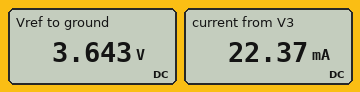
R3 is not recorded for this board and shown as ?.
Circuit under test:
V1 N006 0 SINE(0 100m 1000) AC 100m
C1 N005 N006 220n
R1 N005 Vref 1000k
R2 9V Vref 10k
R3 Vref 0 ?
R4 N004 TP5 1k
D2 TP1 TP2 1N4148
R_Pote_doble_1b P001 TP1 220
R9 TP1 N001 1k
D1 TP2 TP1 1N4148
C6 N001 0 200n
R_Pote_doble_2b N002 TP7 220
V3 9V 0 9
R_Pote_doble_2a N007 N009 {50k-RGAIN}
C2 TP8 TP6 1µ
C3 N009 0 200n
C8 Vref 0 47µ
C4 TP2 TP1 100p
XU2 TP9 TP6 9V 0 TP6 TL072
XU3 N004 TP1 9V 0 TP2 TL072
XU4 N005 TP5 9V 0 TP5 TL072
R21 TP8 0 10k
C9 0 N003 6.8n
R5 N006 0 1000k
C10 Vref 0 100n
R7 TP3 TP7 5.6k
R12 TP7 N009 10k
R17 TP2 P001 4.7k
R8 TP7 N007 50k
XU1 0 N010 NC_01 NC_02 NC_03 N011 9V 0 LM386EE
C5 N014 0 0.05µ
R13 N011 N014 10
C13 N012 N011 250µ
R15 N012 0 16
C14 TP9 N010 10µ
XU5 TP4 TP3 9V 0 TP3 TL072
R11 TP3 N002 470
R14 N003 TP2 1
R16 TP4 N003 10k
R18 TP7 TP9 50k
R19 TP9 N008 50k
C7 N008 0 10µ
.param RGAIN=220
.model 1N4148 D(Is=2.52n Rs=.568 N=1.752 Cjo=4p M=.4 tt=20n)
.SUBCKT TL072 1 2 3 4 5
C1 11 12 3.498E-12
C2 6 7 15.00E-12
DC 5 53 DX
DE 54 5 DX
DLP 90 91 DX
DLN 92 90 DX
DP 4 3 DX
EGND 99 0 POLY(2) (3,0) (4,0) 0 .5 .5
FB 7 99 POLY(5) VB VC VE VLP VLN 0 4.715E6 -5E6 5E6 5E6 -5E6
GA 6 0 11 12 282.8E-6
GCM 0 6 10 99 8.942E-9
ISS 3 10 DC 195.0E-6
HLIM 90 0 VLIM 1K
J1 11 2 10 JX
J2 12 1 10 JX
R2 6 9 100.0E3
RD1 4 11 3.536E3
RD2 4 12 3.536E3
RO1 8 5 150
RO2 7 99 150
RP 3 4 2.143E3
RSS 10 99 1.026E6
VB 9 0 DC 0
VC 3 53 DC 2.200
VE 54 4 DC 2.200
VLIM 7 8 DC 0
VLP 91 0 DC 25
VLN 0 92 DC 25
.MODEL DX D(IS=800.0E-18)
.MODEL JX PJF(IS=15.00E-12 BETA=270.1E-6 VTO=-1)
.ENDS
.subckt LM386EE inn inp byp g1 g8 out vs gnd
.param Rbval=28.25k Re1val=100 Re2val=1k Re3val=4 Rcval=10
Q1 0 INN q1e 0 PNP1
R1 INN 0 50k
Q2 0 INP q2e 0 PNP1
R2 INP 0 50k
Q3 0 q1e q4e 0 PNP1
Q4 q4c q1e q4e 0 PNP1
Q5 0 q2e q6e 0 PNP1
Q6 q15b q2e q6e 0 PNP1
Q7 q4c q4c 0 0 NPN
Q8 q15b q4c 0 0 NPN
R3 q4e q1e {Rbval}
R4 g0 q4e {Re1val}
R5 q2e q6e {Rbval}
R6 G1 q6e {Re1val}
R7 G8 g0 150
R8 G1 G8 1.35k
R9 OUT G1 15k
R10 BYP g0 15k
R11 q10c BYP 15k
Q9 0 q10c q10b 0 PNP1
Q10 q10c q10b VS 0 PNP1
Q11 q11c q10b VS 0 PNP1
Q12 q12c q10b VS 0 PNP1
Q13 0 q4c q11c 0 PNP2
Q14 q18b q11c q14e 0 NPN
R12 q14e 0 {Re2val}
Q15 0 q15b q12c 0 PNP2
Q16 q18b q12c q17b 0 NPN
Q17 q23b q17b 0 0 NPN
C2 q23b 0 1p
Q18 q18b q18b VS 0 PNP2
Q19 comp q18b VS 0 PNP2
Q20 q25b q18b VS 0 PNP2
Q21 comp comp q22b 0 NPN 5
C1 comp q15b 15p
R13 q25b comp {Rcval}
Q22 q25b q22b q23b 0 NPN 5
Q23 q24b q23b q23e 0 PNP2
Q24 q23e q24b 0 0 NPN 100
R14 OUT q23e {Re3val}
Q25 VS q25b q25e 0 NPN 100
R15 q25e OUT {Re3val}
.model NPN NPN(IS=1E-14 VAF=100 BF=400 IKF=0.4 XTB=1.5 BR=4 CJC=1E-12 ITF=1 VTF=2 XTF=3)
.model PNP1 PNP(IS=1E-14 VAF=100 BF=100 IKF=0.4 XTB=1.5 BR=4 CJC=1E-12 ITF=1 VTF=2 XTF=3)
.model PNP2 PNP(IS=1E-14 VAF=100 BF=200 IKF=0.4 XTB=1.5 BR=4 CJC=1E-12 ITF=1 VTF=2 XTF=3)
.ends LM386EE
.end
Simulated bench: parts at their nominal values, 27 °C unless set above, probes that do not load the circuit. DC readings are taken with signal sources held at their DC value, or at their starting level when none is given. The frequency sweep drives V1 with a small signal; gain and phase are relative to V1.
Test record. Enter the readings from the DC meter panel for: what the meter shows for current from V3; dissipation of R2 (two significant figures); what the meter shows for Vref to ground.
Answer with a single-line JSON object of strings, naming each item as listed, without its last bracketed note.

{"what the meter shows for current from V3": "22.37 mA", "dissipation of R2": "2.9 mW", "what the meter shows for Vref to ground": "3.643 V"}
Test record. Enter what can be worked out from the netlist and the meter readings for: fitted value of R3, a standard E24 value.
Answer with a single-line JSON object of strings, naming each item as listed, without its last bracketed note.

{"fitted value of R3, a standard E24 value": "6.8 kΩ"}
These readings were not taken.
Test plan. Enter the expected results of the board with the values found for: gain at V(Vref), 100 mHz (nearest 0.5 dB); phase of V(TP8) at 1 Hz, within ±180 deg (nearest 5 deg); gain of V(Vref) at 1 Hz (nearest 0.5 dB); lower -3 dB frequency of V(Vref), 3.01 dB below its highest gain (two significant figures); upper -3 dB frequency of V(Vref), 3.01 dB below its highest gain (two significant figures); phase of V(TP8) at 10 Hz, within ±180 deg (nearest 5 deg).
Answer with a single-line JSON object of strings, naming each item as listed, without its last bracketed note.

{"gain at V(Vref), 100 mHz": "-65.0 dB", "phase of V(TP8) at 1 Hz, within ±180 deg": "110 deg", "gain of V(Vref) at 1 Hz": "-53.5 dB", "lower -3 dB frequency of V(Vref), 3.01 dB below its highest gain": "320 mHz", "upper -3 dB frequency of V(Vref), 3.01 dB below its highest gain": "1.9 Hz", "phase of V(TP8) at 10 Hz, within ±180 deg": "65 deg"}
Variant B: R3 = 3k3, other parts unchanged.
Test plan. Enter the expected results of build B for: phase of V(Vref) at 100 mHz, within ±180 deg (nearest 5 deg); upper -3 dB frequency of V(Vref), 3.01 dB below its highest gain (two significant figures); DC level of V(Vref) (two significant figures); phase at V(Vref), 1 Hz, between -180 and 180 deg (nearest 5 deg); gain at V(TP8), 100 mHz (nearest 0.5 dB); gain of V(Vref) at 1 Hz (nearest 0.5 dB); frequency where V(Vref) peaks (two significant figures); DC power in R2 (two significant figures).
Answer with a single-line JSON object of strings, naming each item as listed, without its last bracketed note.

{"phase of V(Vref) at 100 mHz, within ±180 deg": "80 deg", "upper -3 dB frequency of V(Vref), 3.01 dB below its highest gain": "2.5 Hz", "DC level of V(Vref)": "2.2 V", "phase at V(Vref), 1 Hz, between -180 and 180 deg": "0 deg", "gain at V(TP8), 100 mHz": "-63.5 dB", "gain of V(Vref) at 1 Hz": "-56.0 dB", "frequency where V(Vref) peaks": "990 mHz", "DC power in R2": "4.6 mW"}
